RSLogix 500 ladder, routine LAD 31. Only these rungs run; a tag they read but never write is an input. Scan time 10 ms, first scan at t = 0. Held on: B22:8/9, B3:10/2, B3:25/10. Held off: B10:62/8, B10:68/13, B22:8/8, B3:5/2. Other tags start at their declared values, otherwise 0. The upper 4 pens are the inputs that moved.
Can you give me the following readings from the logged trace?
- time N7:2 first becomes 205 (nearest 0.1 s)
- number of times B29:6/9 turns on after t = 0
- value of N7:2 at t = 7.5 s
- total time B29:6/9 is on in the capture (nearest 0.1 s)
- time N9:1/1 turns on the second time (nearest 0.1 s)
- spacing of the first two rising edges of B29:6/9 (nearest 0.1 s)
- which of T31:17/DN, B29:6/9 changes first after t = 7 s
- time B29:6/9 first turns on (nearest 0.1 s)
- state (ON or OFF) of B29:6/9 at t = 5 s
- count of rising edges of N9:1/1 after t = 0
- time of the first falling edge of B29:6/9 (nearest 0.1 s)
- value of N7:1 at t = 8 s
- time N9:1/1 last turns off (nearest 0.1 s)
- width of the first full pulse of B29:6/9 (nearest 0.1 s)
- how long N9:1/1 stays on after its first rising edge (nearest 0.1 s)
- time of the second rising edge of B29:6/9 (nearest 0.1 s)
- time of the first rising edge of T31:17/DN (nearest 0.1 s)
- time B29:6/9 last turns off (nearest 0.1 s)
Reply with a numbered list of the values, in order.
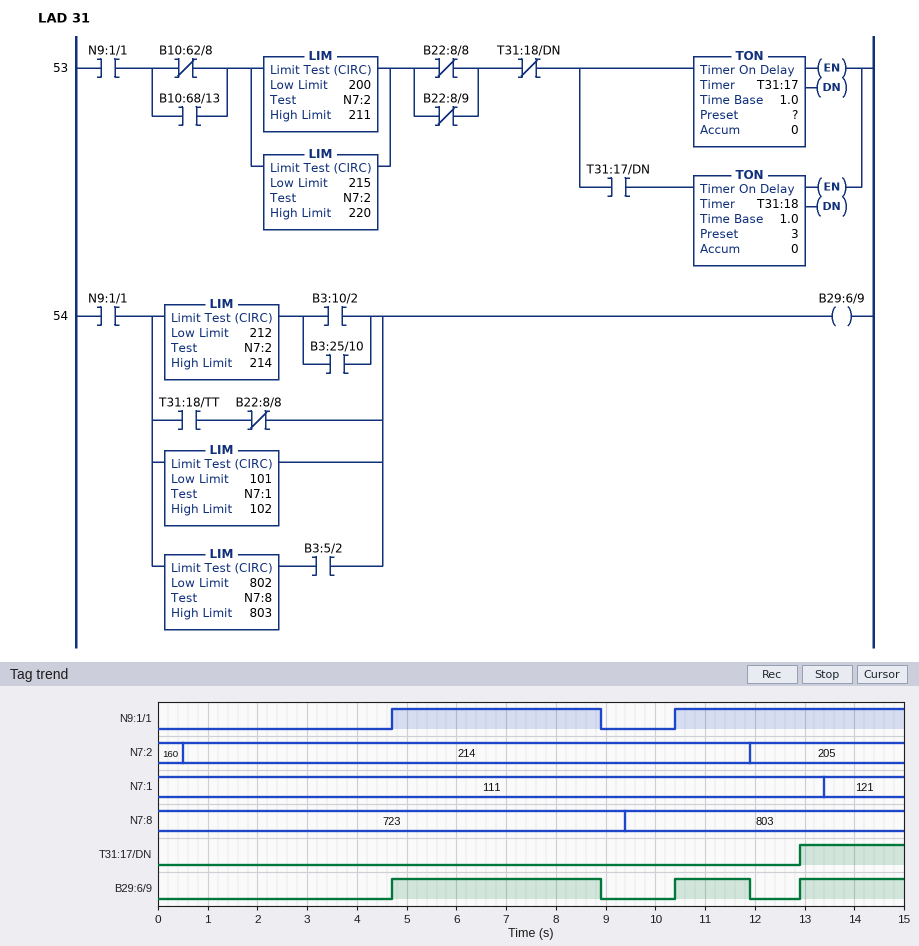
1. 11.9 s
2. 3
3. 214
4. 7.8 s
5. 10.4 s
6. 5.7 s
7. B29:6/9
8. 4.7 s
9. ON
10. 2
11. 8.9 s
12. 111
13. 8.9 s
14. 4.2 s
15. 4.2 s
16. 10.4 s
17. 12.9 s
18. 11.9 s
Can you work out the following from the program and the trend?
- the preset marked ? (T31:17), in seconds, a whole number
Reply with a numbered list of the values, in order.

1. 1 s
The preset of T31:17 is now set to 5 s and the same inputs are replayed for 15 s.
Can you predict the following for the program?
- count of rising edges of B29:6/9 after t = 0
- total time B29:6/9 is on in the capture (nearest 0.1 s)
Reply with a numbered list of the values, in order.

1. 2
2. 5.7 s
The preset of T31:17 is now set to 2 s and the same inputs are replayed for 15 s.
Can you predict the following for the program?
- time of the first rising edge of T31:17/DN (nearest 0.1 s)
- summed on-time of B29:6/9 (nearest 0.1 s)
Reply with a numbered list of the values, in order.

1. 13.9 s
2. 6.8 s
